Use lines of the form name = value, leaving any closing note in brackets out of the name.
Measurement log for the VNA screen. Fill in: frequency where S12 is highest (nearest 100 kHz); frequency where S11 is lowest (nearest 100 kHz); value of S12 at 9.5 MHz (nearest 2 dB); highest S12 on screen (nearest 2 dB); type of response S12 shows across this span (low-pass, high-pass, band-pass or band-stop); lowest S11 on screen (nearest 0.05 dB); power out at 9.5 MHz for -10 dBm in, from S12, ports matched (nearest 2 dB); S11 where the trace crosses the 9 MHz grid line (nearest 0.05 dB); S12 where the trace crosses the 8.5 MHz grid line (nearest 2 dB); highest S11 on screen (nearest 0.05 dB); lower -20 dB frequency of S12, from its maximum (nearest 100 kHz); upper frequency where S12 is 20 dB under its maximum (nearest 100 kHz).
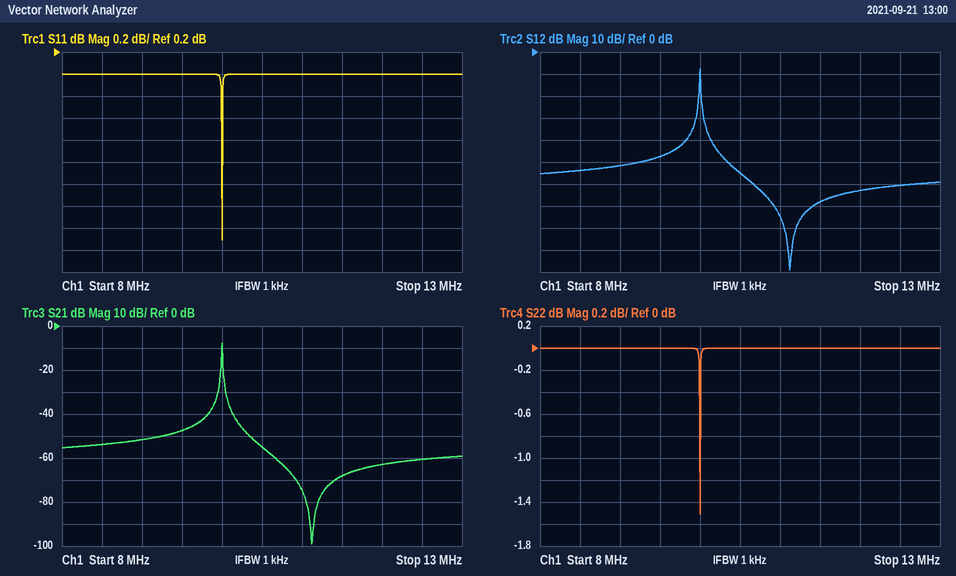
frequency where S12 is highest = 10.0 MHz
frequency where S11 is lowest = 10.0 MHz
value of S12 at 9.5 MHz = -48 dB
highest S12 on screen = -8 dB
type of response S12 shows across this span = band-pass
lowest S11 on screen = -1.50 dB
power out at 9.5 MHz for -10 dBm in, from S12, ports matched = -58 dBm
S11 where the trace crosses the 9 MHz grid line = 0.00 dB
S12 where the trace crosses the 8.5 MHz grid line = -54 dB
highest S11 on screen = 0.00 dB
lower -20 dB frequency of S12, from its maximum = 10.0 MHz
upper frequency where S12 is 20 dB under its maximum = 10.0 MHz
